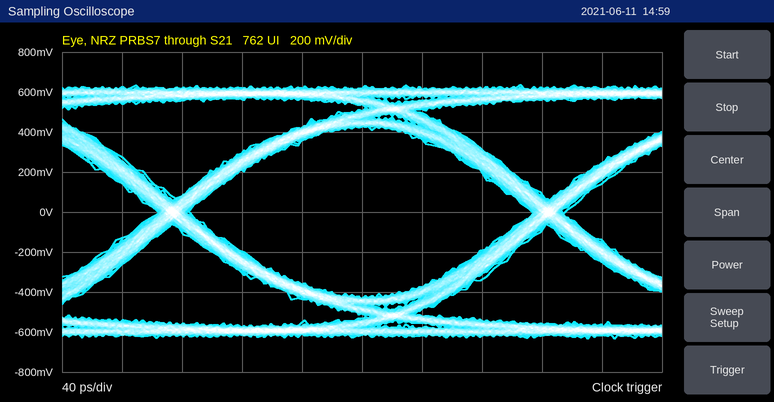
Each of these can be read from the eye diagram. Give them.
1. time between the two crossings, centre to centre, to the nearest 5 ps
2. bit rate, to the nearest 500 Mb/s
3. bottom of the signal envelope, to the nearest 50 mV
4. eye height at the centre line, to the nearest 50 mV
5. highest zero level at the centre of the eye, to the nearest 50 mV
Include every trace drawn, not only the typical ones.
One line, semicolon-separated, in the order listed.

250 ps; 4.0 Gb/s; -650 mV; 850 mV; -450 mV
